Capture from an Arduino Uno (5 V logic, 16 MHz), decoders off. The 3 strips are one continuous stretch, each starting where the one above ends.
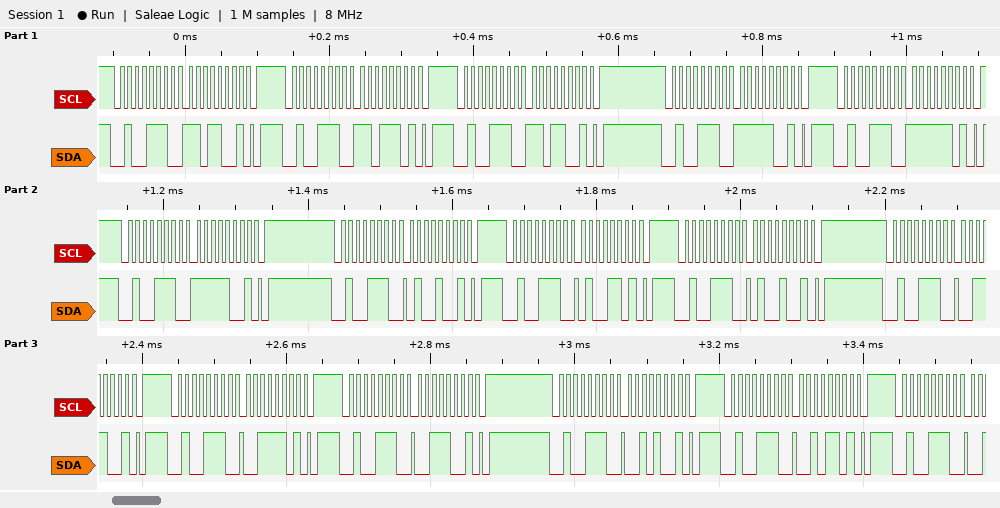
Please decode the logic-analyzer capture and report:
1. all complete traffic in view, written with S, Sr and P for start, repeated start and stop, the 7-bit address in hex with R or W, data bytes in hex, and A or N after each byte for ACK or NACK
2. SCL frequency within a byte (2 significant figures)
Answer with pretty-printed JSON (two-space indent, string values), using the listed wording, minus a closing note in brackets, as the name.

{
  "all complete traffic in view, written with S, Sr and P for start, repeated start and stop, the 7-bit address in hex with R or W, data bytes in hex, and A or N after each byte for ACK or NACK": "S 27W A D9 A P S 27W A DD A P S 27W A D9 A P S 27W A F9 A P S 27W A FD A P S 27W A F9 A P S 27W A 49 A P S 27W A 4D A P S 27W A 49 A P S 27W A 39 A P S 27W A 3D A P S 27W A 39 A P S 27W A 29 A P S 27W A 2D A P S 27W A",
  "SCL frequency within a byte": "100 kHz"
}
